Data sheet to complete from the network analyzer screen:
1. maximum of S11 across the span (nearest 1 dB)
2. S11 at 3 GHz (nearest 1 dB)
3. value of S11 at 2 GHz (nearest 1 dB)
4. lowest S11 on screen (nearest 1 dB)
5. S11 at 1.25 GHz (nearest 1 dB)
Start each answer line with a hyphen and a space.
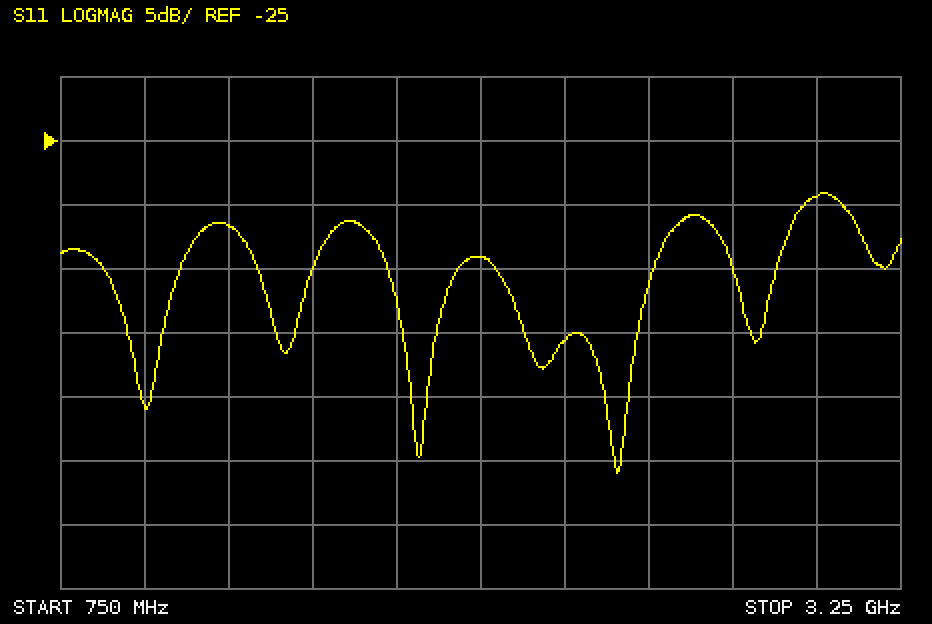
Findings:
- -29 dB
- -29 dB
- -34 dB
- -51 dB
- -32 dB
